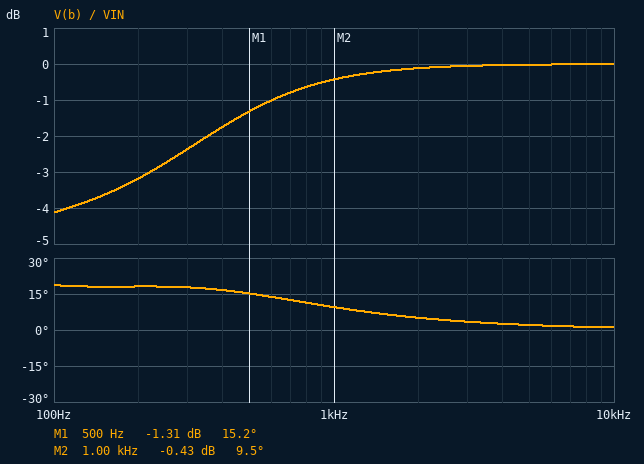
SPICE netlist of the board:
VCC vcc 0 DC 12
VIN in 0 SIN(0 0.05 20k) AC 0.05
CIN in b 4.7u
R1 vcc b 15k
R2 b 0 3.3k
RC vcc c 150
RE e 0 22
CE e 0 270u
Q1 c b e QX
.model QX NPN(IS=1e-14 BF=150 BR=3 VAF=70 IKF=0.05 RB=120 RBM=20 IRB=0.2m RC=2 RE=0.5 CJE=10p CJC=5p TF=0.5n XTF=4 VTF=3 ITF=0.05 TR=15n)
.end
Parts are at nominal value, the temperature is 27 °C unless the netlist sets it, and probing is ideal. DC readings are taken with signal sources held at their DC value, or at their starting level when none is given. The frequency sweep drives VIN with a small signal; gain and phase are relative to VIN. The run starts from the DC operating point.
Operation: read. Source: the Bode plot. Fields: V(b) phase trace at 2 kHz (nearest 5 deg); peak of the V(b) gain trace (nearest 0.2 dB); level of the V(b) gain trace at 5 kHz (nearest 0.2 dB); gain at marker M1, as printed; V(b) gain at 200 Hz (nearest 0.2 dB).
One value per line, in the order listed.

5 deg
0 dB
0 dB
-1.31 dB
-3.2 dB
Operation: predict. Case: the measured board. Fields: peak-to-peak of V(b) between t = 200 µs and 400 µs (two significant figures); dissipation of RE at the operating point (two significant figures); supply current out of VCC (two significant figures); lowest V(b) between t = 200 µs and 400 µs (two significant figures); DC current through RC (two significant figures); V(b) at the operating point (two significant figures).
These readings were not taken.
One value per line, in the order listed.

100 mV
19 mW
30 mA
1.4 V
29 mA
1.4 V
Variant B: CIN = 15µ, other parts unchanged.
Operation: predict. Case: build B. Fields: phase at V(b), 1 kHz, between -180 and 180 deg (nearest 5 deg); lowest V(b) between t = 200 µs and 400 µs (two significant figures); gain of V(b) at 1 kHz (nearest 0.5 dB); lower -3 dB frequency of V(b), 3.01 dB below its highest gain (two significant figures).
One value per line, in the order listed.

5 deg
1.4 V
0 dB
13 Hz
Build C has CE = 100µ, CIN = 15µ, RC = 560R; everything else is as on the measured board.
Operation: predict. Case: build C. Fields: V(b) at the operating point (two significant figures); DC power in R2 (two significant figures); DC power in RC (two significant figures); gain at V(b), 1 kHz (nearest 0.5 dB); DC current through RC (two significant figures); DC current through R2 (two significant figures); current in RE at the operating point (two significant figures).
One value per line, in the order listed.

1.2 V
460 µW
230 mW
0 dB
20 mA
370 µA
21 mA
